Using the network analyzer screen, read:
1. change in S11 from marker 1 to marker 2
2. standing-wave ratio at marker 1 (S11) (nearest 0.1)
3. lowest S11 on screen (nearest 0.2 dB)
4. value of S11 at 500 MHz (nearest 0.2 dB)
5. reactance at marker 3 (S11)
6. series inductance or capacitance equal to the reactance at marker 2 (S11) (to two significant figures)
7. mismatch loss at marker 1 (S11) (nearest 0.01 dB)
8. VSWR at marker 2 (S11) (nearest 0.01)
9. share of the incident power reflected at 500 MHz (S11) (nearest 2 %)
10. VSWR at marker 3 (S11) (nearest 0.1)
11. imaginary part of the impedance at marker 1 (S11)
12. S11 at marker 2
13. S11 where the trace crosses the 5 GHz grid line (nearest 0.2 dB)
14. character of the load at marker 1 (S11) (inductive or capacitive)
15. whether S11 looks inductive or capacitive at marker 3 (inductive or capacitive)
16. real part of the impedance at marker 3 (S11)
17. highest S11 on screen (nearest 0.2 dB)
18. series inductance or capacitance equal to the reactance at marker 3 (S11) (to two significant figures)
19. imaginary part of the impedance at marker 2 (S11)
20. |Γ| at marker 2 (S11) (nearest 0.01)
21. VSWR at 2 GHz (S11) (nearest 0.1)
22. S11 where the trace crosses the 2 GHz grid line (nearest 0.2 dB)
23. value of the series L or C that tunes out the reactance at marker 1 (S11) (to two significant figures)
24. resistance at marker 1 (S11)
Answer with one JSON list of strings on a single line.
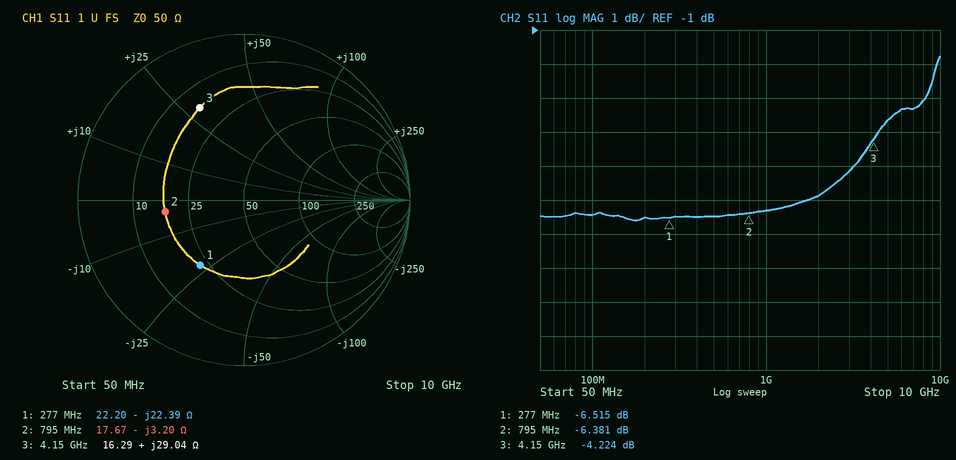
["0.134 dB", "2.8", "-6.6 dB", "-6.4 dB", "+29.04 Ω", "63 pF", "1.10 dB", "2.84", "22 %", "4.2", "-22.39 Ω", "-6.381 dB", "-3.6 dB", "capacitive", "inductive", "16.29 Ω", "-1.8 dB", "1.1 nH", "-3.20 Ω", "0.48", "3.1", "-5.8 dB", "13 nH", "22.20 Ω"]
